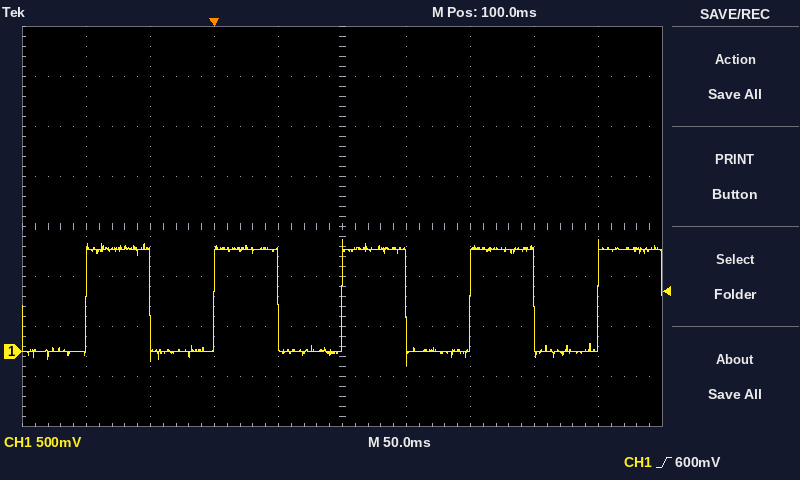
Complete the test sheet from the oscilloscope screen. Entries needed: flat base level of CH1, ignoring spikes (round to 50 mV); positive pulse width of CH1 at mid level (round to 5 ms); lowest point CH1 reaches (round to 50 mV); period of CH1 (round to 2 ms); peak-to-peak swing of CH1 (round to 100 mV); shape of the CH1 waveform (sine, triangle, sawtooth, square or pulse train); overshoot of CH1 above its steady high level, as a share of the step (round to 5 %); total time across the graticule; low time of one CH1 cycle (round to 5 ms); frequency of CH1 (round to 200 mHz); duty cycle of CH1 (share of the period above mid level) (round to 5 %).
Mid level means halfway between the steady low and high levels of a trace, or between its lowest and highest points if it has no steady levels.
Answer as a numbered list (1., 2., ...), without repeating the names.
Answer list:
1. 0 mV
2. 50 ms
3. -150 mV
4. 100 ms
5. 1.30 V
6. square
7. 10 %
8. 500 ms
9. 50 ms
10. 10.0 Hz
11. 50 %
